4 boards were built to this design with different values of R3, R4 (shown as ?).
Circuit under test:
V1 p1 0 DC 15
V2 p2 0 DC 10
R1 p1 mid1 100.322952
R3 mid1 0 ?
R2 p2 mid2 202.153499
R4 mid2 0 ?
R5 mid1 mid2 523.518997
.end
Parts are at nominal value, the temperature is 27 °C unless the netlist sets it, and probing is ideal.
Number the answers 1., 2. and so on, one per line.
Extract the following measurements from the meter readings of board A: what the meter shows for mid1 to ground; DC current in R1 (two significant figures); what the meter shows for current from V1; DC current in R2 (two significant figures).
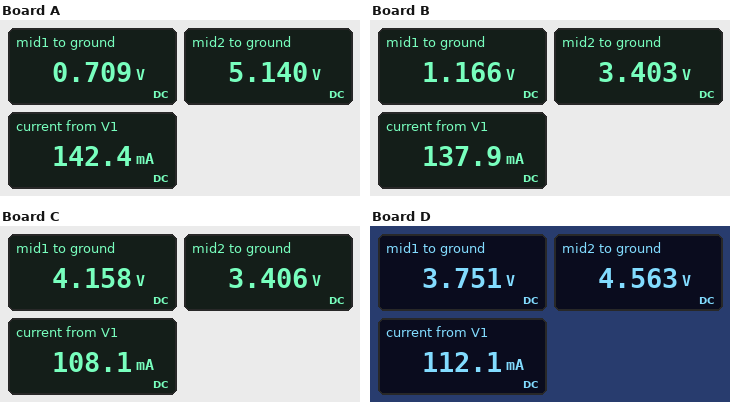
1. 0.709 V
2. 140 mA
3. 142.4 mA
4. 24 mA
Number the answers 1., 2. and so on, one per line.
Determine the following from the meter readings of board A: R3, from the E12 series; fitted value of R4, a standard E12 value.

1. 4.7 Ω
2. 330 Ω
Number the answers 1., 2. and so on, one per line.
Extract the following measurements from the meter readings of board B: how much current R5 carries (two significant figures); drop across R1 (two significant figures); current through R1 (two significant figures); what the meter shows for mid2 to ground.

1. 4.3 mA
2. 14 V
3. 140 mA
4. 3.403 V
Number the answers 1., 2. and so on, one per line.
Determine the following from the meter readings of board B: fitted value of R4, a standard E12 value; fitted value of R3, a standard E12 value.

1. 120 Ω
2. 8.2 Ω
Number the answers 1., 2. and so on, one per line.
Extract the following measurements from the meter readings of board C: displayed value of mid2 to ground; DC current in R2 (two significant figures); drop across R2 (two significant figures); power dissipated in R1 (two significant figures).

1. 3.406 V
2. 33 mA
3. 6.6 V
4. 1.2 W
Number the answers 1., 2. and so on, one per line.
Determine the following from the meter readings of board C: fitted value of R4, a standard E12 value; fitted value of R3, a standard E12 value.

1. 100 Ω
2. 39 Ω
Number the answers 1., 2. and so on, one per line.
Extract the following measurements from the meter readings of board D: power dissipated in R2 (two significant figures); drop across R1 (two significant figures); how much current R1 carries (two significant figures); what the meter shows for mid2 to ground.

1. 150 mW
2. 11 V
3. 110 mA
4. 4.563 V
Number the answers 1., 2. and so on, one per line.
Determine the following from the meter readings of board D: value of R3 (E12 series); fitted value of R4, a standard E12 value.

1. 33 Ω
2. 180 Ω
